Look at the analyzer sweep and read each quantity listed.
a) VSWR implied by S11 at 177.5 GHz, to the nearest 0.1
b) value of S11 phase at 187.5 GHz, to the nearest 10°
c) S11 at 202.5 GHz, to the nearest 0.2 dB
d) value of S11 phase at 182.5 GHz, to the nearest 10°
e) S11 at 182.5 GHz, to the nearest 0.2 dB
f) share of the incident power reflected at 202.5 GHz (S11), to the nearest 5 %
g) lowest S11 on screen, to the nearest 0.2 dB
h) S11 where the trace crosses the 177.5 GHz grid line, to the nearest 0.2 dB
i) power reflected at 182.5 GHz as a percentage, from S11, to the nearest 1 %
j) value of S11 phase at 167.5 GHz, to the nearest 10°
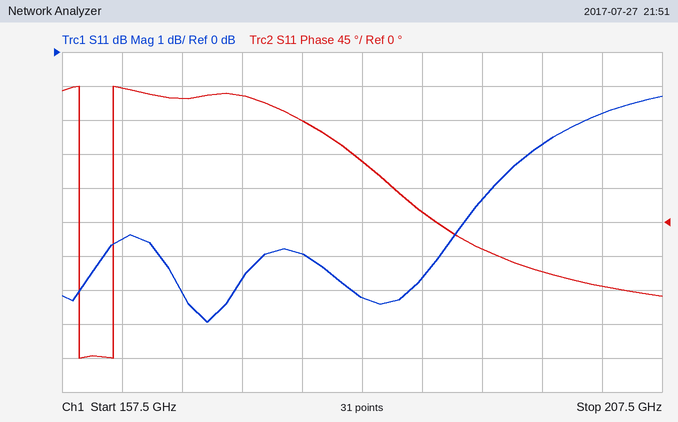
3.0
10°
-1.8 dB
80°
-7.2 dB
65 %
-8.0 dB
-6.0 dB
19 %
160°
